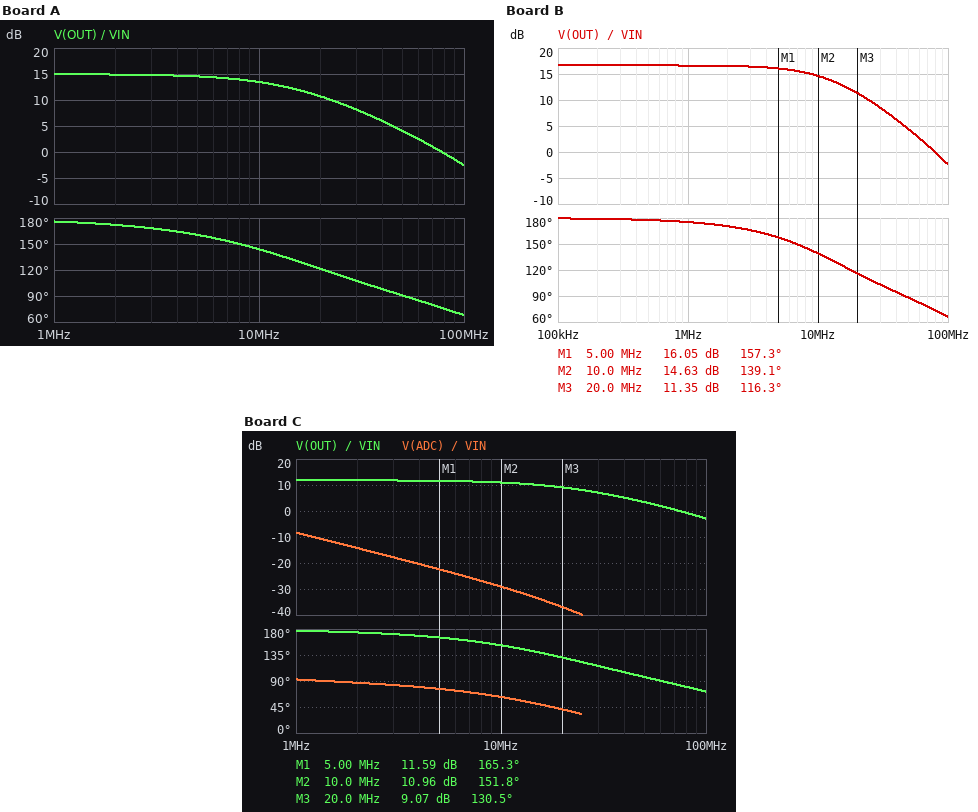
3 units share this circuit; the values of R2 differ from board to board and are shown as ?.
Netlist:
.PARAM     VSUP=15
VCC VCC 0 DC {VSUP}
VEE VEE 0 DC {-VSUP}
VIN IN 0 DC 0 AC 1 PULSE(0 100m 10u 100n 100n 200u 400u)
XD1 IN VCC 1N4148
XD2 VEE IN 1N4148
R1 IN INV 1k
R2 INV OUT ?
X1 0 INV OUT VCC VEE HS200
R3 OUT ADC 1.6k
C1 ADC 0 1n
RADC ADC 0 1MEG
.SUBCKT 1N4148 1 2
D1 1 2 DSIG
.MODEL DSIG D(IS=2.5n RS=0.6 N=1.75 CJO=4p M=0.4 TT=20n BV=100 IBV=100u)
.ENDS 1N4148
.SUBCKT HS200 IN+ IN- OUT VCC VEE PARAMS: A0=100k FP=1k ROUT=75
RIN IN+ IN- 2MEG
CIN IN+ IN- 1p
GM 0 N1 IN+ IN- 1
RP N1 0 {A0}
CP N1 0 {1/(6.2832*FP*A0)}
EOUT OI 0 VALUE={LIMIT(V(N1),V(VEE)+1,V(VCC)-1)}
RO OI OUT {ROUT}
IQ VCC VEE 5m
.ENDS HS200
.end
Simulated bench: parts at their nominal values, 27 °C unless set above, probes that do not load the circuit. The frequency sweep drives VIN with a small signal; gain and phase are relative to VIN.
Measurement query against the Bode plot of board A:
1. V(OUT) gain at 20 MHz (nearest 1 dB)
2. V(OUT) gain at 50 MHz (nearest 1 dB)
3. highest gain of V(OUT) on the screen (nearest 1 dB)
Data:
11 dB
4 dB
15 dB
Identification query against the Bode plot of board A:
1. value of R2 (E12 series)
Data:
5.6 kΩ
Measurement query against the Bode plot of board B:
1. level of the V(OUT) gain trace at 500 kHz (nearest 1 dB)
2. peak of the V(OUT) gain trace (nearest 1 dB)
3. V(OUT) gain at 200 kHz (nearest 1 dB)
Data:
17 dB
17 dB
17 dB
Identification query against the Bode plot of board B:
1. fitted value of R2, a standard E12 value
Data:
6.8 kΩ
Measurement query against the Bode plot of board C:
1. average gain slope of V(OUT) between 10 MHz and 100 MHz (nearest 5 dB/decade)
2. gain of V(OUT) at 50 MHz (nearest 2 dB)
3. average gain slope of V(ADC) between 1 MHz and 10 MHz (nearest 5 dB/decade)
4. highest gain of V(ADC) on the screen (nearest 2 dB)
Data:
-15 dB/decade
4 dB
-20 dB/decade
-8 dB
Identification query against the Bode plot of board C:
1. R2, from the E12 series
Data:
3.9 kΩ
